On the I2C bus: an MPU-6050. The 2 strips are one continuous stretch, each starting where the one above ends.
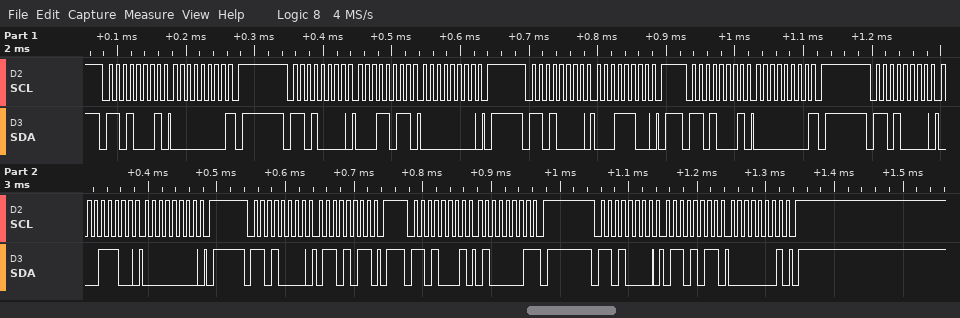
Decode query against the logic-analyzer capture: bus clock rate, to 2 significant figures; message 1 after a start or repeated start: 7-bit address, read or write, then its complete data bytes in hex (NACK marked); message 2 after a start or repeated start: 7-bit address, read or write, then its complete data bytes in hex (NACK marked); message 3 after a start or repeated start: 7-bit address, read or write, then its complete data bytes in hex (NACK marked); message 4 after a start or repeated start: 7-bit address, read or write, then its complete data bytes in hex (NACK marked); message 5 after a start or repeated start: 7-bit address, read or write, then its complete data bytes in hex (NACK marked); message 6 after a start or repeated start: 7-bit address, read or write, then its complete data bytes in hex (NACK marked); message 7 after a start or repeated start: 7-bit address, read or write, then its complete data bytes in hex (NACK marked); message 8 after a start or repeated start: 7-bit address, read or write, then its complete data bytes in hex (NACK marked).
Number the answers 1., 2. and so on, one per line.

1. 100 kHz
2. 0x68 read: 00 NACK
3. 0x68 write: 1B 00
4. 0x68 write: 1C
5. 0x68 read: 00 NACK
6. 0x68 write: 1C 00
7. 0x68 write: 6B
8. 0x68 read: 41 NACK
9. 0x68 write: 6B 01
